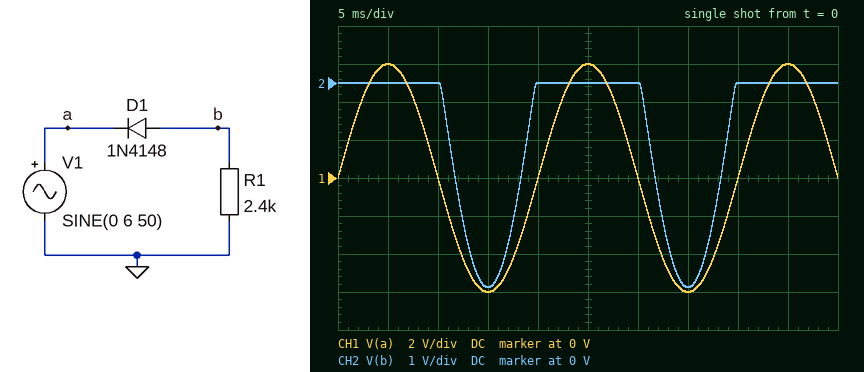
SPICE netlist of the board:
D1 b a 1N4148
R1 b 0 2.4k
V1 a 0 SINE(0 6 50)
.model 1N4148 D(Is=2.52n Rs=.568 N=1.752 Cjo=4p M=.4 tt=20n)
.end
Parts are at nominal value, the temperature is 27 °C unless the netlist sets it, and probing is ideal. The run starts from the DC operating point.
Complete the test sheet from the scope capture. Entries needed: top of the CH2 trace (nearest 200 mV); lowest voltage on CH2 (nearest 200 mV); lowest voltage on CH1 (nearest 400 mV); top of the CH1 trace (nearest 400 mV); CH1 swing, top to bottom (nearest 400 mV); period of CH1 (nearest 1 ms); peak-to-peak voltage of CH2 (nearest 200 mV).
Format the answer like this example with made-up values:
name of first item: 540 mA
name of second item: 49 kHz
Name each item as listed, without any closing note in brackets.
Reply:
top of the CH2 trace: 0 V
lowest voltage on CH2: -5.4 V
lowest voltage on CH1: -6.0 V
top of the CH1 trace: 6.0 V
CH1 swing, top to bottom: 12.0 V
period of CH1: 20 ms
peak-to-peak voltage of CH2: 5.4 V
